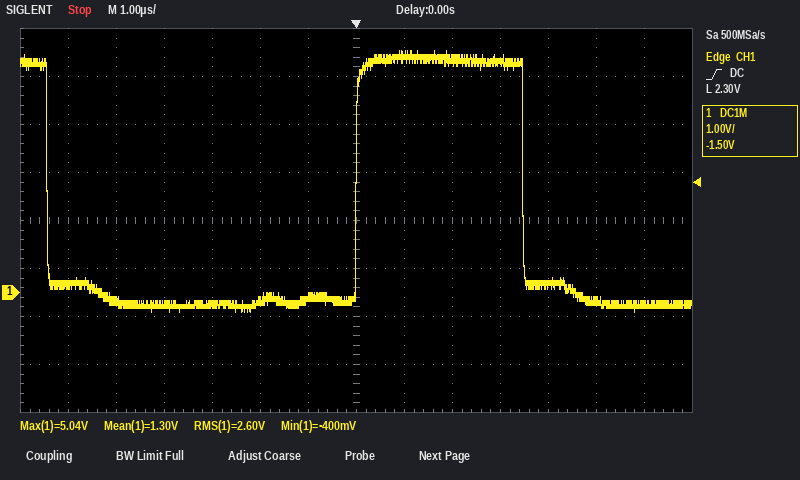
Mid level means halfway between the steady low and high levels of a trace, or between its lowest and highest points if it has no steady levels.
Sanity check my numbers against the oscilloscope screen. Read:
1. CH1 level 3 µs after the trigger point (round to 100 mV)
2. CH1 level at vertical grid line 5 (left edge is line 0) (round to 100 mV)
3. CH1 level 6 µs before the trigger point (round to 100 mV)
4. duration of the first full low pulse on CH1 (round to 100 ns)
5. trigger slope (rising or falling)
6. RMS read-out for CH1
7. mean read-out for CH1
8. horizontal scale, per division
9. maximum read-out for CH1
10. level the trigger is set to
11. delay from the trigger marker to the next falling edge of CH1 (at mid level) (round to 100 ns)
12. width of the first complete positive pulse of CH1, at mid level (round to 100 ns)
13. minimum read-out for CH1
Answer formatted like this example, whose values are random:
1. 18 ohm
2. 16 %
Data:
1. 4.8 V
2. -200 mV
3. 200 mV
4. 6.4 µs
5. rising
6. 2.60 V
7. 1.30 V
8. 1 µs
9. 5.04 V
10. 2.30 V
11. 3.5 µs
12. 3.5 µs
13. -400 mV
